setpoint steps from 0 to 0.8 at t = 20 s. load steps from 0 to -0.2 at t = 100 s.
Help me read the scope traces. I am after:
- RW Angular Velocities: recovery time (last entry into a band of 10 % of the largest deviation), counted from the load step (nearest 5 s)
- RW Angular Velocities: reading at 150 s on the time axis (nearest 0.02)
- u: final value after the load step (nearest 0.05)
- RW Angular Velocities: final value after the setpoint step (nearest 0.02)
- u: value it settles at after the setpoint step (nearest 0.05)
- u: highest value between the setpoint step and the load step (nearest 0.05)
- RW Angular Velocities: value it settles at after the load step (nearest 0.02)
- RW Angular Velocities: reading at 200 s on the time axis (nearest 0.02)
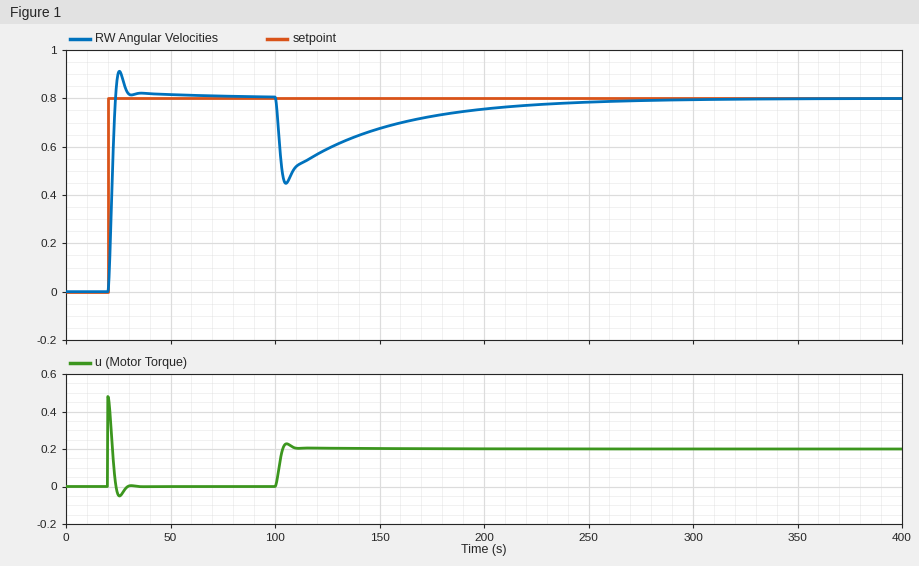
110 s
0.68
0.20
0.80
0.00
0.50
0.80
0.76
